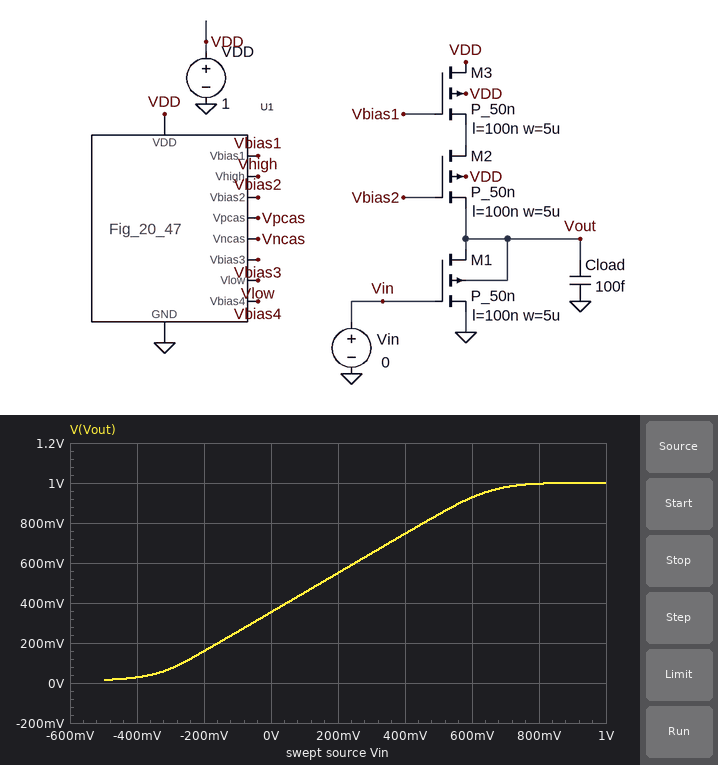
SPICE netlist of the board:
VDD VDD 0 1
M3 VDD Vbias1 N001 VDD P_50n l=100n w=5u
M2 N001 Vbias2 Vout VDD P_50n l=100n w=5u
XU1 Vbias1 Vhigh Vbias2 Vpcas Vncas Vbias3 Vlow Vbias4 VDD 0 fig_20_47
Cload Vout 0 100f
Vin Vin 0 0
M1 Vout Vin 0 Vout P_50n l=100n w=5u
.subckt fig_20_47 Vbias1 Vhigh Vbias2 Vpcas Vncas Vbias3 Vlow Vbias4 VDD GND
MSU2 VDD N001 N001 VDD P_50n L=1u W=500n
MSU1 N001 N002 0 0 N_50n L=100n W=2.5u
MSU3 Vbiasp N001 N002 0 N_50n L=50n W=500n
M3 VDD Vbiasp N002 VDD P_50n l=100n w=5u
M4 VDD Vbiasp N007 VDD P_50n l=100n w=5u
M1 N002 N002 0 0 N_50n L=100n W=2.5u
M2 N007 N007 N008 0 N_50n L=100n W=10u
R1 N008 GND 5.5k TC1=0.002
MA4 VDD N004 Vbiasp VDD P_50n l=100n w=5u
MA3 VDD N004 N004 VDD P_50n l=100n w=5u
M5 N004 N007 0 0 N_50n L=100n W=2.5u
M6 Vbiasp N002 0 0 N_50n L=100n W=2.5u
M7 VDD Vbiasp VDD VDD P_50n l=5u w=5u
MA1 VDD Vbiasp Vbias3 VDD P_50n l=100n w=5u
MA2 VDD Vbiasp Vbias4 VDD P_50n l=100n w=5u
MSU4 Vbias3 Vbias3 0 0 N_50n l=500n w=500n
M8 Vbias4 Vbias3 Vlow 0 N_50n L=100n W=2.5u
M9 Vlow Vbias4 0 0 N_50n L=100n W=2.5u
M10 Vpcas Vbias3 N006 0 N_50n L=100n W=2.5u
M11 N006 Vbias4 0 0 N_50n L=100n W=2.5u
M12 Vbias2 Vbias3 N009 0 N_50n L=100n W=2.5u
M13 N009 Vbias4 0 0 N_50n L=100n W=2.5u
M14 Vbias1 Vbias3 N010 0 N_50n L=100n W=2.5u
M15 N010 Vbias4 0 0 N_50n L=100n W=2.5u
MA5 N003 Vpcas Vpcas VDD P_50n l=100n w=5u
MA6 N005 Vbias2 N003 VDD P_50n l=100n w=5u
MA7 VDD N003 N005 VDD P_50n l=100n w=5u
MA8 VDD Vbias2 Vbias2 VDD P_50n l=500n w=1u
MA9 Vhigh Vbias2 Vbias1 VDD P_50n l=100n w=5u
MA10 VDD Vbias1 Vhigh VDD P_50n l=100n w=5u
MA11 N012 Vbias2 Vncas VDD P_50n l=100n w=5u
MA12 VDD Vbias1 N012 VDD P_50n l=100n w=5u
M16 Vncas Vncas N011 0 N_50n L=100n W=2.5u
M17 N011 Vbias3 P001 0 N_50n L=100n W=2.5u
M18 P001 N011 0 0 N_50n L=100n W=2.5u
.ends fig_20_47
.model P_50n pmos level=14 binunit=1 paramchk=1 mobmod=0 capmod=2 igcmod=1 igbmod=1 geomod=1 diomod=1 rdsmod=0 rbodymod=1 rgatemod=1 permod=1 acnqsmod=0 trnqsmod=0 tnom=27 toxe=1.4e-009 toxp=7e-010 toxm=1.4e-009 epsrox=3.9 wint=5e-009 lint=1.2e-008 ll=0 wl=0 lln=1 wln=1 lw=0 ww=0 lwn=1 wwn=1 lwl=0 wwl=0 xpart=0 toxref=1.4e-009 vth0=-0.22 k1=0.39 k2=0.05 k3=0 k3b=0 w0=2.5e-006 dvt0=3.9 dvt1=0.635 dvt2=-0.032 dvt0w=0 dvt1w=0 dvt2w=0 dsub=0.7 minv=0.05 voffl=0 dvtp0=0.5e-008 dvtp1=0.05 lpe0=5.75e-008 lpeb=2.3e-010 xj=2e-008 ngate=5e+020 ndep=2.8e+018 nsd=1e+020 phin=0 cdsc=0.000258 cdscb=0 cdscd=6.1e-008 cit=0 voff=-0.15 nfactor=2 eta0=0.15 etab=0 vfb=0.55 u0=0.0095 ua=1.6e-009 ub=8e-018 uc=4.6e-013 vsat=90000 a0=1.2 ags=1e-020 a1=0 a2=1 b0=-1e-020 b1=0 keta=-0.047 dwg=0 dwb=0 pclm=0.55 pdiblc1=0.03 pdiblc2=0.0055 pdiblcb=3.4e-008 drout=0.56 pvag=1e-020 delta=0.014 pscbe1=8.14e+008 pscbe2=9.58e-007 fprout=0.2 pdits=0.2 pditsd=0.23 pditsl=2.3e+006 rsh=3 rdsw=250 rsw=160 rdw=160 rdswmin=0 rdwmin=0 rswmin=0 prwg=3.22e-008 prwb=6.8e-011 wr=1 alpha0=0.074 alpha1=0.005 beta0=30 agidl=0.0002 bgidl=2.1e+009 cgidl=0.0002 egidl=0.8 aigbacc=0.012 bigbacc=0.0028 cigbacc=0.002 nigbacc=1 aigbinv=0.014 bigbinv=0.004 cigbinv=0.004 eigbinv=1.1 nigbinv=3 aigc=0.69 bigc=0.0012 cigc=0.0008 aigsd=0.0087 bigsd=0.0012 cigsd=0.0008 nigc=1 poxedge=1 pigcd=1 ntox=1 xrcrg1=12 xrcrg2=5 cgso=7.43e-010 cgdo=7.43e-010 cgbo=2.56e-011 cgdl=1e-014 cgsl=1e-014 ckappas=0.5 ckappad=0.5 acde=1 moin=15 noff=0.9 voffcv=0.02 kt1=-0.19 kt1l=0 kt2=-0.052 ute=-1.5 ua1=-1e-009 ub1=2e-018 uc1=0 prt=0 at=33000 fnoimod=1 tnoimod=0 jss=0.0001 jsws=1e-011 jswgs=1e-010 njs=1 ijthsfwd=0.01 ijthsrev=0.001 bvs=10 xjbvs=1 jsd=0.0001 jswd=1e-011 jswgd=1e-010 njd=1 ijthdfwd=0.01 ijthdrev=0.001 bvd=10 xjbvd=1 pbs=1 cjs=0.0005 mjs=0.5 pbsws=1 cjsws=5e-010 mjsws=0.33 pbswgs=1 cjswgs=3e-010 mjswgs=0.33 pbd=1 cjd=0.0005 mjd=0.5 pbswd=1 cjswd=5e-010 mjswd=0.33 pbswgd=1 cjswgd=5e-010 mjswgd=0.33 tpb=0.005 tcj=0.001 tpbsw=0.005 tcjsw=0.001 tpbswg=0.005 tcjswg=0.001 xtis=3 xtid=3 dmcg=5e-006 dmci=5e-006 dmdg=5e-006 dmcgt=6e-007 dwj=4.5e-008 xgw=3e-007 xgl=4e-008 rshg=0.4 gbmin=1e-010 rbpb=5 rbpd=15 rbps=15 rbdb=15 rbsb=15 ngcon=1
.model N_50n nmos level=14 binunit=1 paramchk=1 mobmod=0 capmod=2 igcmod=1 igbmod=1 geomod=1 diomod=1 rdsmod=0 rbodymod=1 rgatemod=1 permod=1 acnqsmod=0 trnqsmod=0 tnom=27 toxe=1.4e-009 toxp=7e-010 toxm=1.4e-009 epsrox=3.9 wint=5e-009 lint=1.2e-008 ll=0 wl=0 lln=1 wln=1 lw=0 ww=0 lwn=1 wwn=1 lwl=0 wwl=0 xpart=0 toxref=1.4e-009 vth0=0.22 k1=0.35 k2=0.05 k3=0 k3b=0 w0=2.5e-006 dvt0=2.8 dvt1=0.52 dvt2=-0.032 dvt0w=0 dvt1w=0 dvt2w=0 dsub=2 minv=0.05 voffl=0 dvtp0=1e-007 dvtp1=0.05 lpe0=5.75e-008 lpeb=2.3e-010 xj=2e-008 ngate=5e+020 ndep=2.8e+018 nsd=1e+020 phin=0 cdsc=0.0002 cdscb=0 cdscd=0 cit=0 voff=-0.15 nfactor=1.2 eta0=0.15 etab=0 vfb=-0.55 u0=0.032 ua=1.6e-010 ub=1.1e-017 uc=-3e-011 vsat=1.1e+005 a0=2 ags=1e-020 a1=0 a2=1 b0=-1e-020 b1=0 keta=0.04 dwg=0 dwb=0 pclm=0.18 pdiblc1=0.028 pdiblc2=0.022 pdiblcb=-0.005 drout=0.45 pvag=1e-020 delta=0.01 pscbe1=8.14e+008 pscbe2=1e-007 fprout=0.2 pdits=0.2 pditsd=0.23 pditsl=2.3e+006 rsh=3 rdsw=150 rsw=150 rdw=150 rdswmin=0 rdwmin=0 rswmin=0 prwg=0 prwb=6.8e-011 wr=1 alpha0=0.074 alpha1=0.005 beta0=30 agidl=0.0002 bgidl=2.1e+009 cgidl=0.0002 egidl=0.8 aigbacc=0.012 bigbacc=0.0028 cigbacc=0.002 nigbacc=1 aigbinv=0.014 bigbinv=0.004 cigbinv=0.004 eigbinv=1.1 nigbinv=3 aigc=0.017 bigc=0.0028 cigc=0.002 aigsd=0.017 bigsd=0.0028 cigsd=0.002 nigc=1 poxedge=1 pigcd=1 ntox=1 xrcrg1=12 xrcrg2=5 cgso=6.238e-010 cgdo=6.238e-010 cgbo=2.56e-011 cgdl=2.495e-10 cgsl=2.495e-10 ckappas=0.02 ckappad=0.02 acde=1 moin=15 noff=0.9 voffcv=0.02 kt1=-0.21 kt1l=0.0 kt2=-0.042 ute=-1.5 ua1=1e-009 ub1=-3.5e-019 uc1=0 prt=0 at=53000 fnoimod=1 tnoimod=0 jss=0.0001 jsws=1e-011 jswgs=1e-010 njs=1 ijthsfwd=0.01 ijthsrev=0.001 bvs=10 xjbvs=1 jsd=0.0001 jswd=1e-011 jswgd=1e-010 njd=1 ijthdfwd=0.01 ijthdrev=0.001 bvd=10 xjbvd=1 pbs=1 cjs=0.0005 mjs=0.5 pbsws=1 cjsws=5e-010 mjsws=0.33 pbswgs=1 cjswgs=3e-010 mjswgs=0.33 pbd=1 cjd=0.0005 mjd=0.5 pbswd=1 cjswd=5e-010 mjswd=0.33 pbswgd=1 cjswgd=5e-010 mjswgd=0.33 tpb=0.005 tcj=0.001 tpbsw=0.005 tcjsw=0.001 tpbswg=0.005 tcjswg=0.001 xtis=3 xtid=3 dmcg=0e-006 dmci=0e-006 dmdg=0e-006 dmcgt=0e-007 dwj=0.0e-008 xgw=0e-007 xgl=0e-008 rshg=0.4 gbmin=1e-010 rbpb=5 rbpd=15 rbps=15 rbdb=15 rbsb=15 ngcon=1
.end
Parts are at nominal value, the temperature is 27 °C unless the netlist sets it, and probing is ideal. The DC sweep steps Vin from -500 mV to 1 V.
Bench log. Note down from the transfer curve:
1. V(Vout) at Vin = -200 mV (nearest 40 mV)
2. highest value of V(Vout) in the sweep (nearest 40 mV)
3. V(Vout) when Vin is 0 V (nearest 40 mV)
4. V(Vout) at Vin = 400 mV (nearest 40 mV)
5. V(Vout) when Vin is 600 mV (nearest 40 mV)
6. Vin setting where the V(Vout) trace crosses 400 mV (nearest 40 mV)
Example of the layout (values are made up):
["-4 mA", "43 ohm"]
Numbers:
["160 mV", "1.00 V", "360 mV", "760 mV", "920 mV", "40 mV"]
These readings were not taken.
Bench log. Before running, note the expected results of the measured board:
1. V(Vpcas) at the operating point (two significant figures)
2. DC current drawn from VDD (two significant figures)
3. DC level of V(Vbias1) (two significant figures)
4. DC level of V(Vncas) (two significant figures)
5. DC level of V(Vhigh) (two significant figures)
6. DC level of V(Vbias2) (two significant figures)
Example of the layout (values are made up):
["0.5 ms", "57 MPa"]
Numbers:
["200 mV", "120 µA", "640 mV", "800 mV", "790 mV", "370 mV"]
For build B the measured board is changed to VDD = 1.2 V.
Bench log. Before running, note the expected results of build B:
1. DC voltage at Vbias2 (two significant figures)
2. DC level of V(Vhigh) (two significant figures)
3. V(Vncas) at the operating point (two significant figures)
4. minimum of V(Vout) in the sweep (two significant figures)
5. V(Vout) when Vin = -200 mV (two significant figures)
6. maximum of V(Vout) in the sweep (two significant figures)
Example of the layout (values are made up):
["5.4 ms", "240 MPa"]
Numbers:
["560 mV", "980 mV", "810 mV", "16 mV", "160 mV", "1.2 V"]
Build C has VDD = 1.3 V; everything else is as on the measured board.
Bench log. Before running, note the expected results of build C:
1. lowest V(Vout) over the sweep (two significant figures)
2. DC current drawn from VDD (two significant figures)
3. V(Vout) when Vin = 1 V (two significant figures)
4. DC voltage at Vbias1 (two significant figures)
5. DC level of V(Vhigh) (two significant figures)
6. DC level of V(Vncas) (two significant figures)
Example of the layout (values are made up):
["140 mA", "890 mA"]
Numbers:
["16 mV", "130 µA", "1.3 V", "940 mV", "1.1 V", "810 mV"]
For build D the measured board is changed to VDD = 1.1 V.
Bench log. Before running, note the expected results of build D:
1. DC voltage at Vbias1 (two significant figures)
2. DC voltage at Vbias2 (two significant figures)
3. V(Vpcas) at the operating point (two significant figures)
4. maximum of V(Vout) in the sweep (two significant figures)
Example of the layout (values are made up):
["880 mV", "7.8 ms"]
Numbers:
["740 mV", "460 mV", "290 mV", "1.1 V"]
